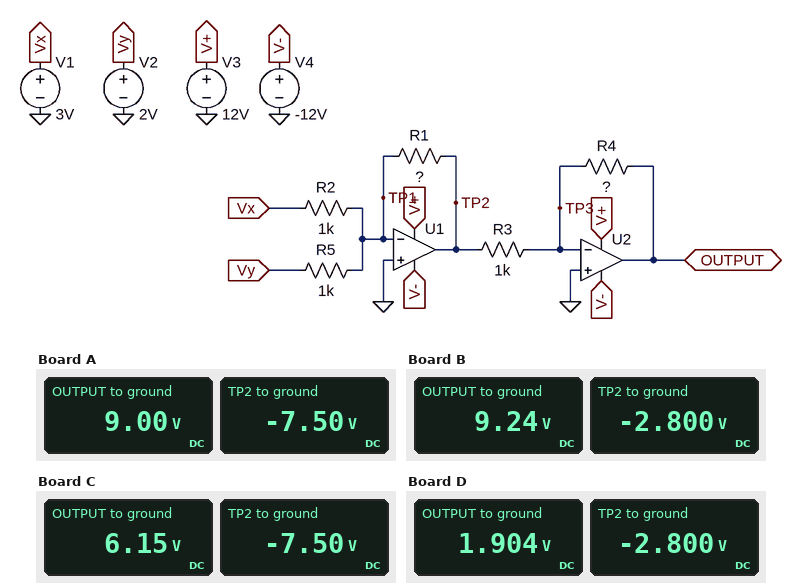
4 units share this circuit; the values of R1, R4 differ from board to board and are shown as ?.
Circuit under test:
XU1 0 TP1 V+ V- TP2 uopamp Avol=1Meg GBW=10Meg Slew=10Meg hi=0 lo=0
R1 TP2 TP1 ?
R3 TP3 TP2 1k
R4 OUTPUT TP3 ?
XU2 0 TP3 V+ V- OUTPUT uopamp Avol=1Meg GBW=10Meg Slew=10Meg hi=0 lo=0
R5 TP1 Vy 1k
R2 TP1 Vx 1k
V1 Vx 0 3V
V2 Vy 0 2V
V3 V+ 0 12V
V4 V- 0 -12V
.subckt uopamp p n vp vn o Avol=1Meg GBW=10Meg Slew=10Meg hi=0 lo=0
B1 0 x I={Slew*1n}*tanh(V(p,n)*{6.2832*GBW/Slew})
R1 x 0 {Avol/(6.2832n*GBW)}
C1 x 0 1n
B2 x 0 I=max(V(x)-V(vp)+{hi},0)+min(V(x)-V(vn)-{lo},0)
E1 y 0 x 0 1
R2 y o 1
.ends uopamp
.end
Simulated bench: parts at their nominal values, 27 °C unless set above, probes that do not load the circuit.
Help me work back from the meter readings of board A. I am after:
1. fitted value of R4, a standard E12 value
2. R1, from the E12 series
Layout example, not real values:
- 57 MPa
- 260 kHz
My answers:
- 1.2 kΩ
- 1.5 kΩ
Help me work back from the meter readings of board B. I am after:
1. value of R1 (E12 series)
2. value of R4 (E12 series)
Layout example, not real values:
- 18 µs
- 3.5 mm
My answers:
- 560 Ω
- 3.3 kΩ
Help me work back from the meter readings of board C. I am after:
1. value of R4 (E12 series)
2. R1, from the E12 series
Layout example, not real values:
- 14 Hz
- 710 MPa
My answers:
- 820 Ω
- 1.5 kΩ
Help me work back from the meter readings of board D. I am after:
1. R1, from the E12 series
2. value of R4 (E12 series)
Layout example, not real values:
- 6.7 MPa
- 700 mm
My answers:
- 560 Ω
- 680 Ω
